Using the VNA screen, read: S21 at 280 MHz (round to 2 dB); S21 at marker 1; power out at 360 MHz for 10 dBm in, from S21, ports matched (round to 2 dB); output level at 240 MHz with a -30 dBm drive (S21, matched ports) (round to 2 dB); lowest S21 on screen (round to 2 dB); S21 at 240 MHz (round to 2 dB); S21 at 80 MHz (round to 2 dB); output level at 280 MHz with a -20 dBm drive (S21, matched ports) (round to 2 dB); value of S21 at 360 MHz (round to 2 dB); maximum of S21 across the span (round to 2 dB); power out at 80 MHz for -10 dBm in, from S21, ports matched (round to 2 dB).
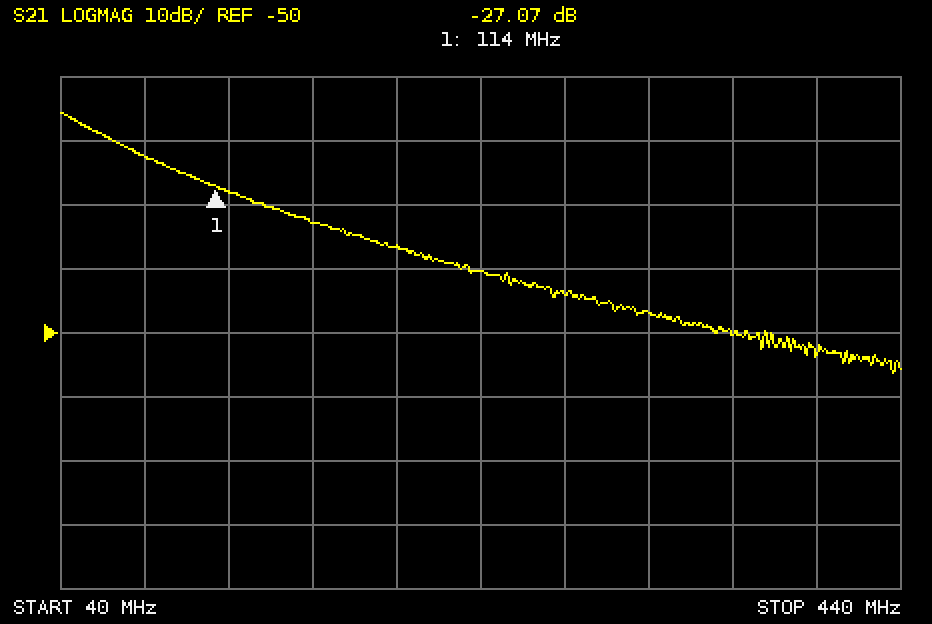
-44 dB
-27.07 dB
-40 dBm
-70 dBm
-56 dB
-40 dB
-22 dB
-64 dBm
-50 dB
-16 dB
-32 dBm
